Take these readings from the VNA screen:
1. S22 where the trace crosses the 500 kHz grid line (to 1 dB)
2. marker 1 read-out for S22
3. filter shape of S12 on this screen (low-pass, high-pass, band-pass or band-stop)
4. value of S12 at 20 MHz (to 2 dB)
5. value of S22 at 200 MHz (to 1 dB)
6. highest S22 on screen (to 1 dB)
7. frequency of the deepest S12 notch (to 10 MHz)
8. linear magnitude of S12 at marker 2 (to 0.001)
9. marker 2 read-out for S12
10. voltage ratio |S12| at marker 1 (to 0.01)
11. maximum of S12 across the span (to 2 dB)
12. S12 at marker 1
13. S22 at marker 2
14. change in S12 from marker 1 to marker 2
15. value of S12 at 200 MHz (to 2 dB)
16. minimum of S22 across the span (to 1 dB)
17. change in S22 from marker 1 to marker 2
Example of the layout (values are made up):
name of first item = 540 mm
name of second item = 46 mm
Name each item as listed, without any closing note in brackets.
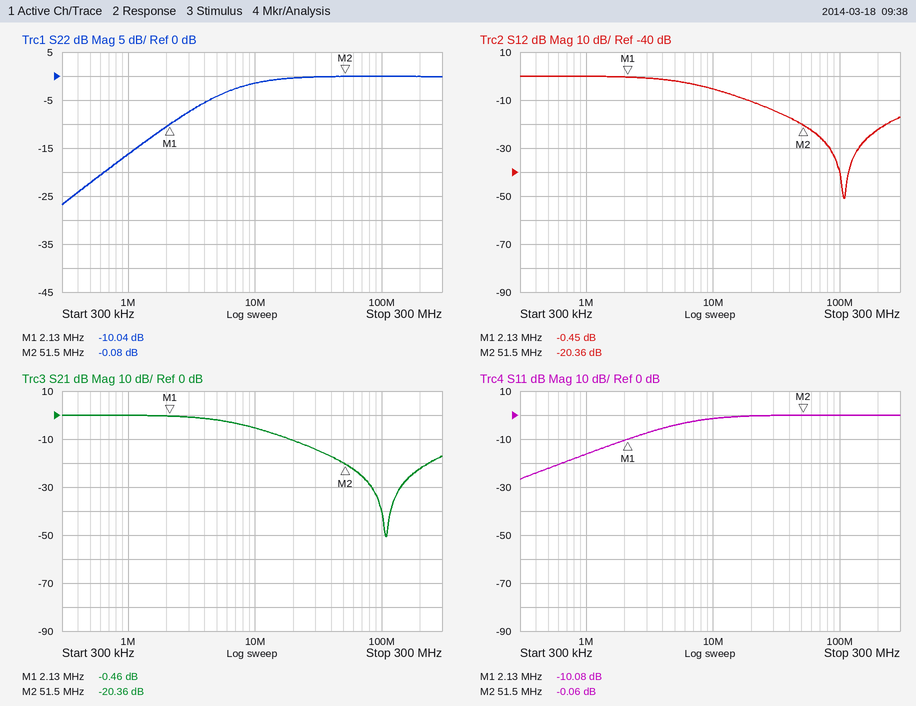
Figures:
S22 where the trace crosses the 500 kHz grid line = -22 dB
marker 1 read-out for S22 = -10.04 dB
filter shape of S12 on this screen = low-pass
value of S12 at 20 MHz = -10 dB
value of S22 at 200 MHz = 0 dB
highest S22 on screen = 0 dB
frequency of the deepest S12 notch = 110 MHz
linear magnitude of S12 at marker 2 = 0.096
marker 2 read-out for S12 = -20.36 dB
voltage ratio |S12| at marker 1 = 0.95
maximum of S12 across the span = 0 dB
S12 at marker 1 = -0.45 dB
S22 at marker 2 = -0.08 dB
change in S12 from marker 1 to marker 2 = -19.91 dB
value of S12 at 200 MHz = -22 dB
minimum of S22 across the span = -27 dB
change in S22 from marker 1 to marker 2 = 9.96 dB
